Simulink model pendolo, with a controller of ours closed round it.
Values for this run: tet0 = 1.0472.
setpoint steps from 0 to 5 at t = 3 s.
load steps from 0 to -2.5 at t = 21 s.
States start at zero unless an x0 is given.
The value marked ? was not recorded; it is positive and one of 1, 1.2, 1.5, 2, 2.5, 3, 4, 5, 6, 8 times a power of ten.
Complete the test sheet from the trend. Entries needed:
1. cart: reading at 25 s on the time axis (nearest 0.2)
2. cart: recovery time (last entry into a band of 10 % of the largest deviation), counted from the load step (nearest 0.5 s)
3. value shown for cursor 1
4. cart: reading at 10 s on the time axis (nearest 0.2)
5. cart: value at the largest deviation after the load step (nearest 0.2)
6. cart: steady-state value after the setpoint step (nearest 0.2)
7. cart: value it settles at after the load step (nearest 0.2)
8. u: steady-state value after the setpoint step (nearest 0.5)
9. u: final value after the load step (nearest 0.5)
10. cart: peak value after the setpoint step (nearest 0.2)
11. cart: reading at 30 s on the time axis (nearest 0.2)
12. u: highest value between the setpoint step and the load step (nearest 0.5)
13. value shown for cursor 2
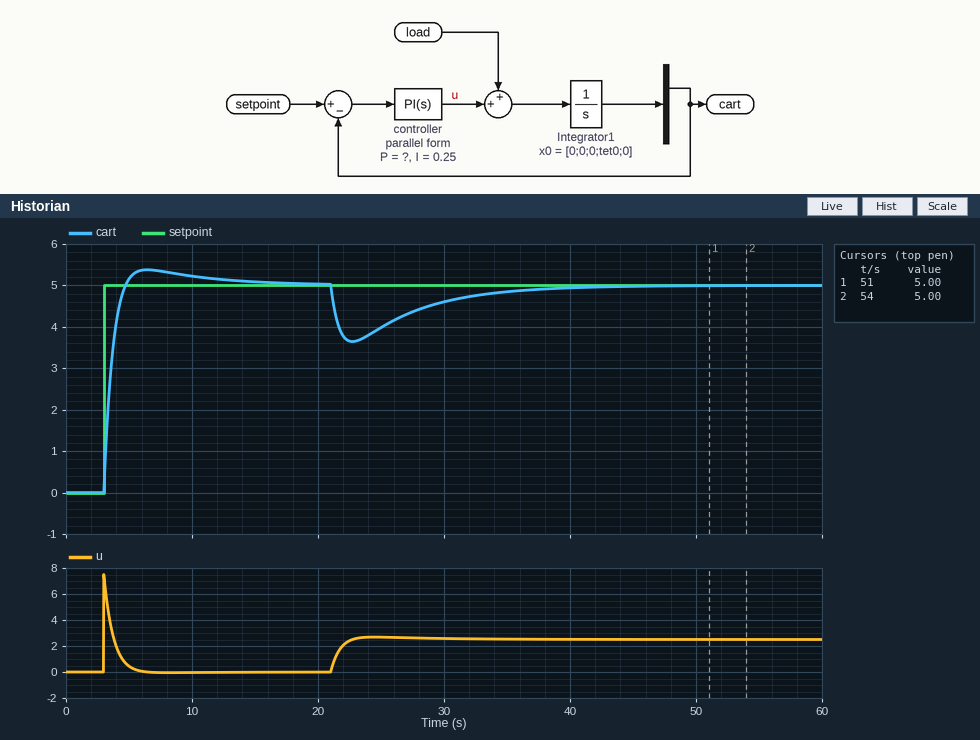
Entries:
4.0
14.5 s
5.00
5.2
3.6
5.0
5.0
0.0
2.5
5.4
4.6
7.5
5.00
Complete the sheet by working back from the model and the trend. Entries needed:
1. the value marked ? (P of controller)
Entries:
1.5
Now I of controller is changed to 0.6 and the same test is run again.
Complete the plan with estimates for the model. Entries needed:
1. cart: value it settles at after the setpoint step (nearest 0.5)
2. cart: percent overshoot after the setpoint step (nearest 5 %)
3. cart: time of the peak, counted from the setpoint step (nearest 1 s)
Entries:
5.0
15 %
3 s
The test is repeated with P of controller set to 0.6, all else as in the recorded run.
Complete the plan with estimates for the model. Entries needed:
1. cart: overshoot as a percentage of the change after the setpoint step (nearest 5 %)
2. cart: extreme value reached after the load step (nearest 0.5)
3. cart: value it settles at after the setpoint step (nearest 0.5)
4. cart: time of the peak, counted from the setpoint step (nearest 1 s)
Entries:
25 %
2.5
5.0
5 s
